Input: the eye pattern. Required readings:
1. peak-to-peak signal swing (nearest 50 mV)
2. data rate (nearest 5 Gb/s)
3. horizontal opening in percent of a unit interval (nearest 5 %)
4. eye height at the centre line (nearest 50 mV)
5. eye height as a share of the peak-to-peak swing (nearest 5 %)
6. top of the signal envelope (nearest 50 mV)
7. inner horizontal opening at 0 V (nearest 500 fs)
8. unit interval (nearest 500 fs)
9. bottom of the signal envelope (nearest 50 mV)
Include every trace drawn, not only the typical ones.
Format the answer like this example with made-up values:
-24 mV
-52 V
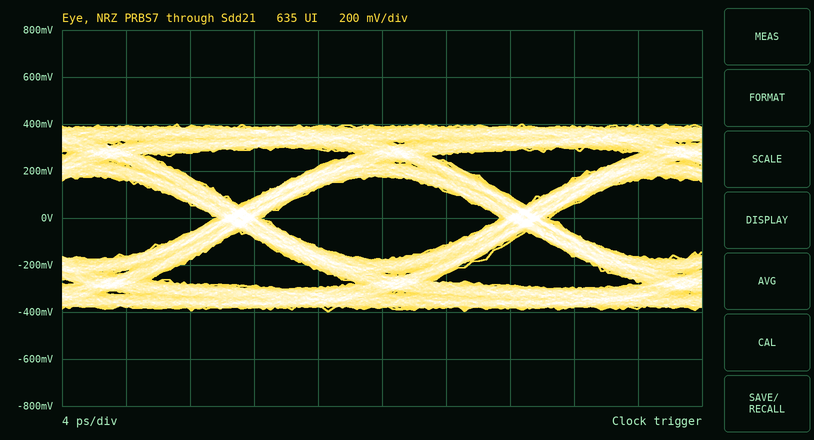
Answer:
800 mV
55 Gb/s
85 %
350 mV
45 %
400 mV
15.0 ps
18.0 ps
-400 mV
